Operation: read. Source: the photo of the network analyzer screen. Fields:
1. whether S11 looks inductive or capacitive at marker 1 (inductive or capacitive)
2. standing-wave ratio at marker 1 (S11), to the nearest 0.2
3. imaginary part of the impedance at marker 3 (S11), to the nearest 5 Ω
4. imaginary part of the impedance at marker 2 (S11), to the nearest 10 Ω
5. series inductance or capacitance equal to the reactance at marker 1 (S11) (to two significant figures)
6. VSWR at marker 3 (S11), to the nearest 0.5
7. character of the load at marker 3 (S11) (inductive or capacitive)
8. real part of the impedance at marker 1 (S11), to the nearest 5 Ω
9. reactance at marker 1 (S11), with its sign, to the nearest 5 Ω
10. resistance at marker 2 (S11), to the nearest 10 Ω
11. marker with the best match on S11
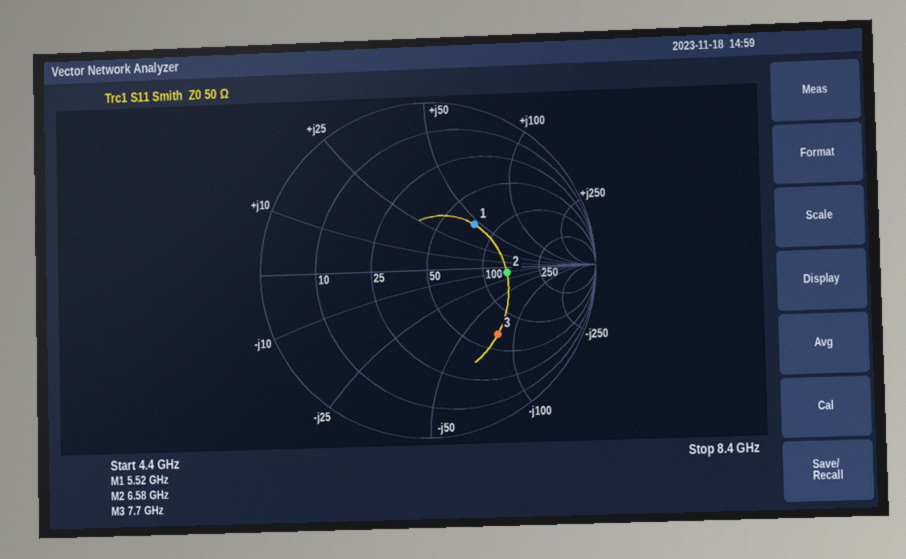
inductive
2.2
-80 Ω
-10 Ω
1.3 nH
3.5
capacitive
75 Ω
+45 Ω
140 Ω
marker 1
